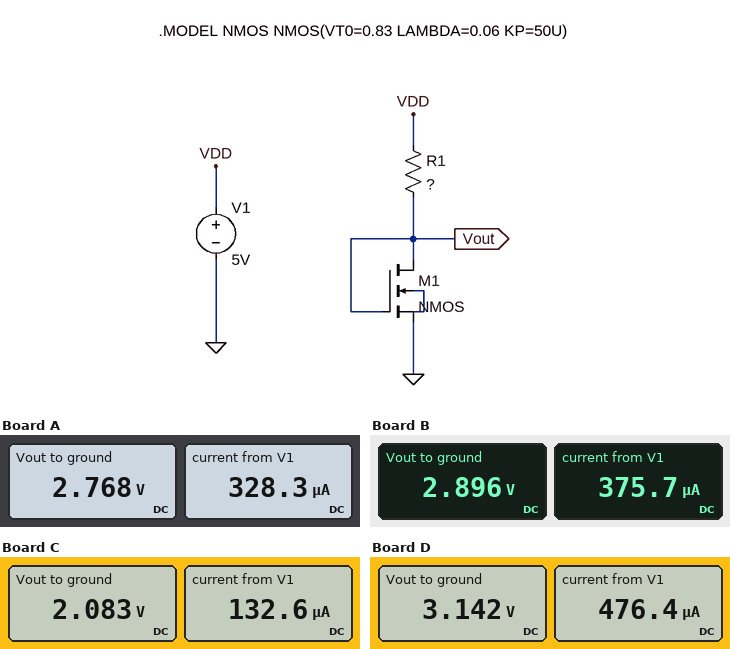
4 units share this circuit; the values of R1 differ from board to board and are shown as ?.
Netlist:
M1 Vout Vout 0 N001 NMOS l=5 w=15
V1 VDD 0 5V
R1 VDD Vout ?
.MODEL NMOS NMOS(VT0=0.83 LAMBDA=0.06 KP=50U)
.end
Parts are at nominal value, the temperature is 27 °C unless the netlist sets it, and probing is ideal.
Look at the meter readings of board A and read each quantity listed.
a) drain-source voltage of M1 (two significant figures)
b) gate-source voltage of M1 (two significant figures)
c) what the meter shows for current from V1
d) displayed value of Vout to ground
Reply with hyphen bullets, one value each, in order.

- 2.8 V
- 2.8 V
- 328.3 µA
- 2.768 V
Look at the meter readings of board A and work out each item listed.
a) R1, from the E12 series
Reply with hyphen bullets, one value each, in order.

- 6.8 kΩ
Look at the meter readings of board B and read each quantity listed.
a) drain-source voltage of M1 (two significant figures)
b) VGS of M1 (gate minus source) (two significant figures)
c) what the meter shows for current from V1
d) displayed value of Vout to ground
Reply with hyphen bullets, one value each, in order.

- 2.9 V
- 2.9 V
- 375.7 µA
- 2.896 V
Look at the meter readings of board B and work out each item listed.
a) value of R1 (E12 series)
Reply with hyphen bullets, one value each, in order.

- 5.6 kΩ
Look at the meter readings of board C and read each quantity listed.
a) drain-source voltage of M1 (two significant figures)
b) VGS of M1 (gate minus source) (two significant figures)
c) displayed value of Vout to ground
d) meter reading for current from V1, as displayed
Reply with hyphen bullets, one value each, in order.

- 2.1 V
- 2.1 V
- 2.083 V
- 132.6 µA
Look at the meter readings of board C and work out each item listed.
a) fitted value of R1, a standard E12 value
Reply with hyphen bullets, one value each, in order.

- 22 kΩ
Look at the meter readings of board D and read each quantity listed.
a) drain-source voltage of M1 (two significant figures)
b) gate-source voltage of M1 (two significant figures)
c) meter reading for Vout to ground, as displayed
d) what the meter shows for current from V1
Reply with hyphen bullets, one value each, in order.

- 3.1 V
- 3.1 V
- 3.142 V
- 476.4 µA
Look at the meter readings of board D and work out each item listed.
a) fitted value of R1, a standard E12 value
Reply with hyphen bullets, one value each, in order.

- 3.9 kΩ
